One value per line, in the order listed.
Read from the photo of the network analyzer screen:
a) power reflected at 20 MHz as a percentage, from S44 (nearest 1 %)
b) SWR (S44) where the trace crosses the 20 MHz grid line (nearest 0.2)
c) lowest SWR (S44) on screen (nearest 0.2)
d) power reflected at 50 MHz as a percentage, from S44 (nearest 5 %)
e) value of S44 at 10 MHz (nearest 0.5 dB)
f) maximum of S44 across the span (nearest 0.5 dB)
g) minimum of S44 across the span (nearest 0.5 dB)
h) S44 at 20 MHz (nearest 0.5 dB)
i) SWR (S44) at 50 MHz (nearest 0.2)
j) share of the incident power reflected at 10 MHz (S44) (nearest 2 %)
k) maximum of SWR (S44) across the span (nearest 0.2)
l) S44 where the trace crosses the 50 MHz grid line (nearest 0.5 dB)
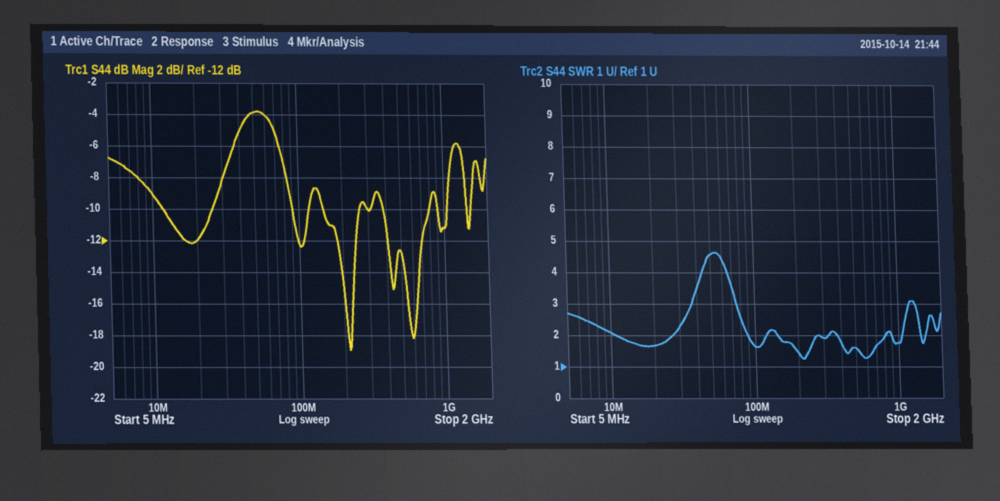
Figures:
6 %
1.6
1.2
40 %
-9.0 dB
-4.0 dB
-19.0 dB
-12.0 dB
4.6
12 %
4.6
-4.0 dB
